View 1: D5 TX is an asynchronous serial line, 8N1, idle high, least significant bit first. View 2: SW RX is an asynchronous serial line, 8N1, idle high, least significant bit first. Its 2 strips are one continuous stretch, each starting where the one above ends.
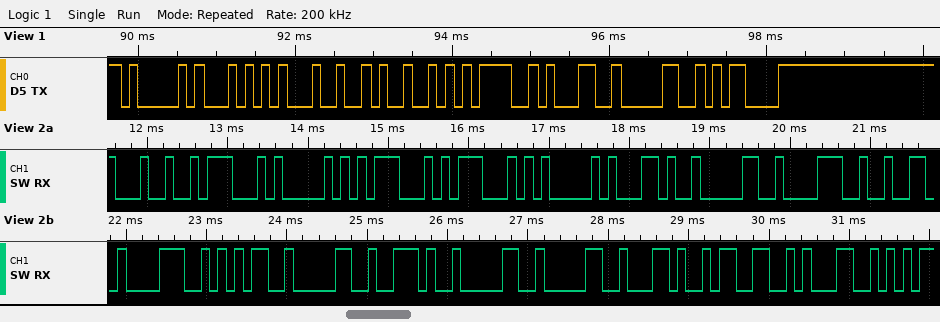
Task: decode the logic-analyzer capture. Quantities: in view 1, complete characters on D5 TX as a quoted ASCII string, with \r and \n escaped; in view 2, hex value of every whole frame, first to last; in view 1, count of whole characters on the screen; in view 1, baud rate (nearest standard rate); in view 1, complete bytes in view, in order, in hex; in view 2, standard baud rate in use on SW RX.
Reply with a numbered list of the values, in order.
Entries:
1. "AT$I=10\r"
2. 24 47 50 47 47 41 2C 30 38 32 38 35 30 2E 30 30 2C 33 31
3. 8
4. 9600 baud
5. 41 54 24 49 3D 31 30 0D
6. 9600 baud
